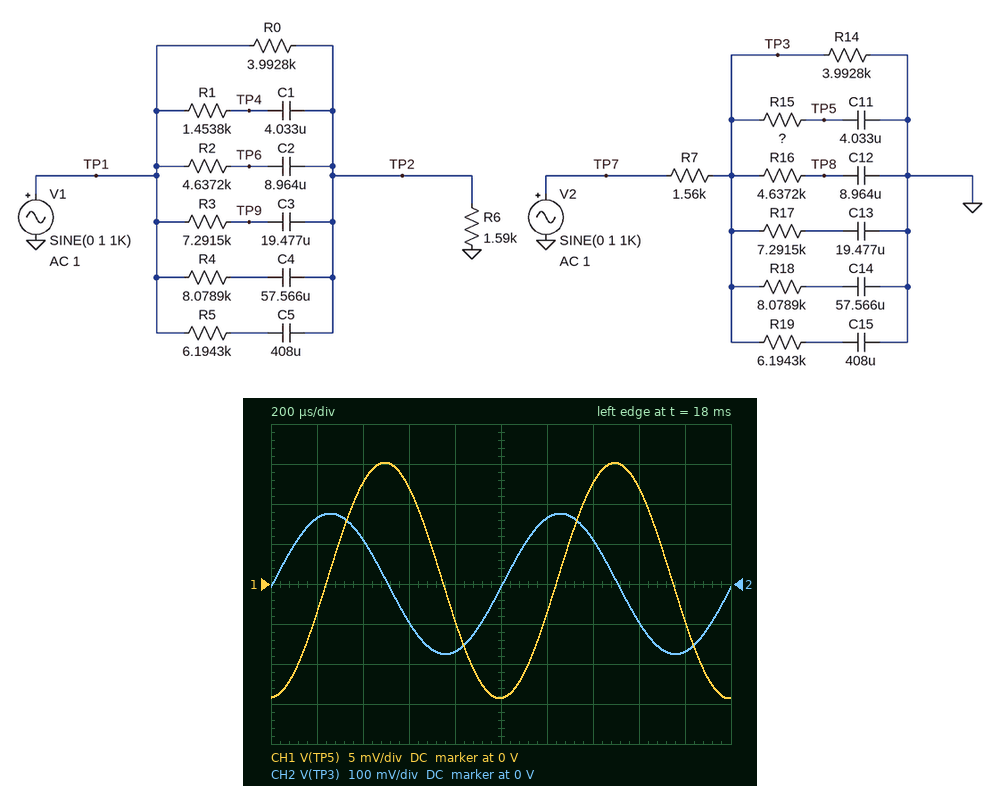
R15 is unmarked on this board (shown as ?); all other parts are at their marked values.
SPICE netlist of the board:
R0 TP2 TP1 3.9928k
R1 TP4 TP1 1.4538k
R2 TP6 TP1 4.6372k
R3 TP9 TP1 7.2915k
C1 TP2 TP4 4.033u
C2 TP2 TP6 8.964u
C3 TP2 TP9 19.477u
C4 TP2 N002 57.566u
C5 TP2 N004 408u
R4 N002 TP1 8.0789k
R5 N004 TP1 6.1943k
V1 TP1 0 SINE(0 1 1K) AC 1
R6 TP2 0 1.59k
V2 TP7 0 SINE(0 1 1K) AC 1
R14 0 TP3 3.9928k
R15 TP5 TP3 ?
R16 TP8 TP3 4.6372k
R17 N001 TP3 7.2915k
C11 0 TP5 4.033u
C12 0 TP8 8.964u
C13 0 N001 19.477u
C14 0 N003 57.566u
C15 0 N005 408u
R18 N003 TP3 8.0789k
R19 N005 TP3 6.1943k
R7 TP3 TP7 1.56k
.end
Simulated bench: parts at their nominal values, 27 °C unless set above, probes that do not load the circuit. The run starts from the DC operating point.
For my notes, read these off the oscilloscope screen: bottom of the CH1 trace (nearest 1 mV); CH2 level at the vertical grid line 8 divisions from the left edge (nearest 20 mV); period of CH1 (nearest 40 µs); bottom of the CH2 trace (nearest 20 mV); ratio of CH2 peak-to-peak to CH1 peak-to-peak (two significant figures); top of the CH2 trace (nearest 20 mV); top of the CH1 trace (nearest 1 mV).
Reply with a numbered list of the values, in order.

1. -14 mV
2. -100 mV
3. 1.00 ms
4. -180 mV
5. 12
6. 180 mV
7. 15 mV
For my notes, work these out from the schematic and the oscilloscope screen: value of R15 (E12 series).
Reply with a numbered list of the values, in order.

1. 470 Ω
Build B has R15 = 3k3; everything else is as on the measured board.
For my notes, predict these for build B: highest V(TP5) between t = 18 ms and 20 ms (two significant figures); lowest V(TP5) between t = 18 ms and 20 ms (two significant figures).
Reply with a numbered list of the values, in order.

1. 5.6 mV
2. -2.8 mV
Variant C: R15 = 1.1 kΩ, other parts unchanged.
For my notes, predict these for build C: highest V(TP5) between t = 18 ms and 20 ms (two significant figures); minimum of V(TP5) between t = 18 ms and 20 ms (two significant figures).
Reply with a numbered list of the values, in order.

1. 10 mV
2. -8.7 mV
